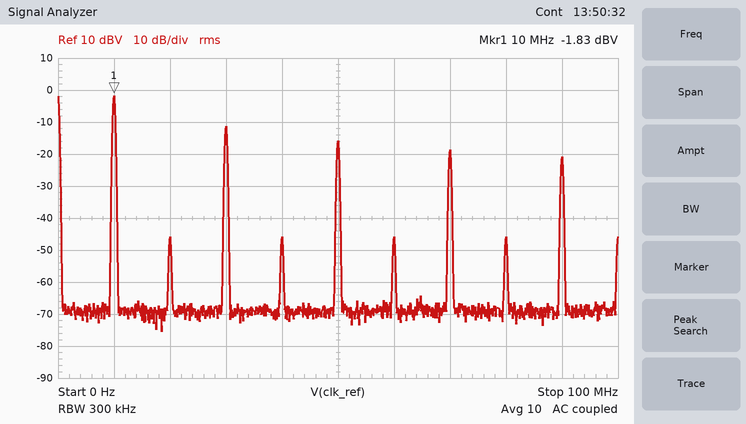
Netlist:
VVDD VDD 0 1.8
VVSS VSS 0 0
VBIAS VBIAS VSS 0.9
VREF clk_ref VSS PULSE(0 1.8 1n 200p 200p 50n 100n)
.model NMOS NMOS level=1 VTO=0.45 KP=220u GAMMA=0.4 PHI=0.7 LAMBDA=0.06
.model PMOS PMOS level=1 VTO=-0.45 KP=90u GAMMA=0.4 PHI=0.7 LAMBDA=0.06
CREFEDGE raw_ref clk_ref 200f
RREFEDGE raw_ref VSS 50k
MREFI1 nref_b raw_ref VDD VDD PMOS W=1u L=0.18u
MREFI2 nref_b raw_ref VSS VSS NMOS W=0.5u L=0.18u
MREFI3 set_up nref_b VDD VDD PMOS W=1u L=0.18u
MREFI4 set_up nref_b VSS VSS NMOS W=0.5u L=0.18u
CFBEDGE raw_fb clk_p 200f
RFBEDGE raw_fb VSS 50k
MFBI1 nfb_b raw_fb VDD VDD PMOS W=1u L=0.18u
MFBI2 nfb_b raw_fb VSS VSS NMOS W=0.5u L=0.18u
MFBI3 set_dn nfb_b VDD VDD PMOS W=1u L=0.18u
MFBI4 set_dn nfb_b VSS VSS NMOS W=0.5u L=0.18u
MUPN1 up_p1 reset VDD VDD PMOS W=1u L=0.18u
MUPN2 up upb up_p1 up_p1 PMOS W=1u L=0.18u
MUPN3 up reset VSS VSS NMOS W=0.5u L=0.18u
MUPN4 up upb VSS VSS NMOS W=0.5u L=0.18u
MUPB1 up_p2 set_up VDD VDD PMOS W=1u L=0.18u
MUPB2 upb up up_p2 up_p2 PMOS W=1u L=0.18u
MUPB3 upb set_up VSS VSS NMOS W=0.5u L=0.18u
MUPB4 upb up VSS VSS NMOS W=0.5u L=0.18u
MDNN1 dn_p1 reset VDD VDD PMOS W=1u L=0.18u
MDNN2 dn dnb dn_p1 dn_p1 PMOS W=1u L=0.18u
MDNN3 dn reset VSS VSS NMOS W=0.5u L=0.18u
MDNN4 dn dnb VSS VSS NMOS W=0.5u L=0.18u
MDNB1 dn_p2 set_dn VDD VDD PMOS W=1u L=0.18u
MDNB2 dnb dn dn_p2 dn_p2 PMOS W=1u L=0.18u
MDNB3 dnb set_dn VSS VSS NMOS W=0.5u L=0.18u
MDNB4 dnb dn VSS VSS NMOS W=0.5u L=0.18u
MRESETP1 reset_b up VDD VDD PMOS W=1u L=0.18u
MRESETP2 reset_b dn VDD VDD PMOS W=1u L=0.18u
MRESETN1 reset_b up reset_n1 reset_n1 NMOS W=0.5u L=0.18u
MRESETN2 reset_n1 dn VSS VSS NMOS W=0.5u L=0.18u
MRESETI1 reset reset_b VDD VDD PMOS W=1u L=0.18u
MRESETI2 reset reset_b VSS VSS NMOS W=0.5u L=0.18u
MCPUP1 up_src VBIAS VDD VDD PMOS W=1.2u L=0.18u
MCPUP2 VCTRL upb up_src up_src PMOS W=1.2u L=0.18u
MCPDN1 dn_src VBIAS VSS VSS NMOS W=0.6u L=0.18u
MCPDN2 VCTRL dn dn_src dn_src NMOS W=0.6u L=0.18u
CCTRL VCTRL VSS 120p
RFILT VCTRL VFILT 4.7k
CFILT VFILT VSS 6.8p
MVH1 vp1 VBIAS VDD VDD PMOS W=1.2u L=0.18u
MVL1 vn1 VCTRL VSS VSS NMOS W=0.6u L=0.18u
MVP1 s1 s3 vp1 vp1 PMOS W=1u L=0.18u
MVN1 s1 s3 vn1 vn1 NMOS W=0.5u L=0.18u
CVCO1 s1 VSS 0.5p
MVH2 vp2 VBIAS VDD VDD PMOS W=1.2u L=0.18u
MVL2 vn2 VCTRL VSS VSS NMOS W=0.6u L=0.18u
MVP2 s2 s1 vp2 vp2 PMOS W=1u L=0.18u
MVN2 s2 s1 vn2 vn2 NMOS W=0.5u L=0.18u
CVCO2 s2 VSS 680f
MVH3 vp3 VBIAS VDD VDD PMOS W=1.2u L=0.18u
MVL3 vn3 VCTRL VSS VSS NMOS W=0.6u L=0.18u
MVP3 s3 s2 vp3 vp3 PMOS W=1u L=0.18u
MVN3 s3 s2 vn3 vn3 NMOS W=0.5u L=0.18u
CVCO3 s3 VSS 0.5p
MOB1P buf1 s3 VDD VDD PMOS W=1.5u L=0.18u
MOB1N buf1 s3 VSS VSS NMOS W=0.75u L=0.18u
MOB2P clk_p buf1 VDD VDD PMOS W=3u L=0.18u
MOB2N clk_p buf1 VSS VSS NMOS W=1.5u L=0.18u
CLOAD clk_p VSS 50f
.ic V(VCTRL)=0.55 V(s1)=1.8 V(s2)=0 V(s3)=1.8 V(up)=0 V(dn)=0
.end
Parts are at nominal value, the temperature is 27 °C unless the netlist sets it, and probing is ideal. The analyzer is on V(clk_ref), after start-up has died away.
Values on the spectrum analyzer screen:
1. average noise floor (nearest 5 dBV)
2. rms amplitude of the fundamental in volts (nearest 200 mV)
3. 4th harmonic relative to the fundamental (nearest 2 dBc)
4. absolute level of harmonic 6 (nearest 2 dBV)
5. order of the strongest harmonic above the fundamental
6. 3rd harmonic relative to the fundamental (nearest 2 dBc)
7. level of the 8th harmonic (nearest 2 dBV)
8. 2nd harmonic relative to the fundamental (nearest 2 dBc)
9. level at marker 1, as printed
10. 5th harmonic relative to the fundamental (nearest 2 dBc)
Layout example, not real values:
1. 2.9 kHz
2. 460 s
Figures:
1. -70 dBV
2. 800 mV
3. -44 dBc
4. -46 dBV
5. 3
6. -10 dBc
7. -46 dBV
8. -44 dBc
9. -1.83 dBV
10. -14 dBc
